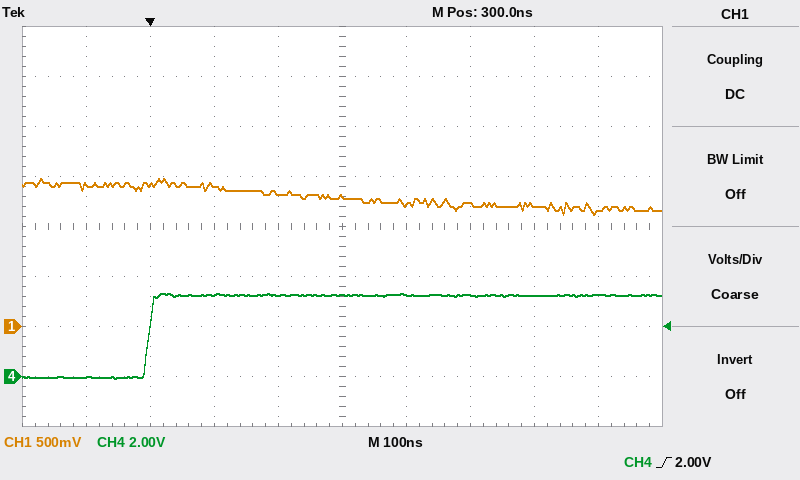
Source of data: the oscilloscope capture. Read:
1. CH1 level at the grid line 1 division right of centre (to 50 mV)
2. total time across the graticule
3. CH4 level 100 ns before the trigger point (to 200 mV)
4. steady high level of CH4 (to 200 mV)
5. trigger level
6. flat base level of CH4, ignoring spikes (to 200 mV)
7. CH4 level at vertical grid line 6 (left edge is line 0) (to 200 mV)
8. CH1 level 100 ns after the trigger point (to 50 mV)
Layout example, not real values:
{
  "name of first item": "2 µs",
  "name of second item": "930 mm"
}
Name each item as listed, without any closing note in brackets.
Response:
{
  "CH1 level at the grid line 1 division right of centre": "1.20 V",
  "total time across the graticule": "1 µs",
  "CH4 level 100 ns before the trigger point": "0.0 V",
  "steady high level of CH4": "3.2 V",
  "trigger level": "2.00 V",
  "flat base level of CH4, ignoring spikes": "0.0 V",
  "CH4 level at vertical grid line 6 (left edge is line 0)": "3.2 V",
  "CH1 level 100 ns after the trigger point": "1.40 V"
}
